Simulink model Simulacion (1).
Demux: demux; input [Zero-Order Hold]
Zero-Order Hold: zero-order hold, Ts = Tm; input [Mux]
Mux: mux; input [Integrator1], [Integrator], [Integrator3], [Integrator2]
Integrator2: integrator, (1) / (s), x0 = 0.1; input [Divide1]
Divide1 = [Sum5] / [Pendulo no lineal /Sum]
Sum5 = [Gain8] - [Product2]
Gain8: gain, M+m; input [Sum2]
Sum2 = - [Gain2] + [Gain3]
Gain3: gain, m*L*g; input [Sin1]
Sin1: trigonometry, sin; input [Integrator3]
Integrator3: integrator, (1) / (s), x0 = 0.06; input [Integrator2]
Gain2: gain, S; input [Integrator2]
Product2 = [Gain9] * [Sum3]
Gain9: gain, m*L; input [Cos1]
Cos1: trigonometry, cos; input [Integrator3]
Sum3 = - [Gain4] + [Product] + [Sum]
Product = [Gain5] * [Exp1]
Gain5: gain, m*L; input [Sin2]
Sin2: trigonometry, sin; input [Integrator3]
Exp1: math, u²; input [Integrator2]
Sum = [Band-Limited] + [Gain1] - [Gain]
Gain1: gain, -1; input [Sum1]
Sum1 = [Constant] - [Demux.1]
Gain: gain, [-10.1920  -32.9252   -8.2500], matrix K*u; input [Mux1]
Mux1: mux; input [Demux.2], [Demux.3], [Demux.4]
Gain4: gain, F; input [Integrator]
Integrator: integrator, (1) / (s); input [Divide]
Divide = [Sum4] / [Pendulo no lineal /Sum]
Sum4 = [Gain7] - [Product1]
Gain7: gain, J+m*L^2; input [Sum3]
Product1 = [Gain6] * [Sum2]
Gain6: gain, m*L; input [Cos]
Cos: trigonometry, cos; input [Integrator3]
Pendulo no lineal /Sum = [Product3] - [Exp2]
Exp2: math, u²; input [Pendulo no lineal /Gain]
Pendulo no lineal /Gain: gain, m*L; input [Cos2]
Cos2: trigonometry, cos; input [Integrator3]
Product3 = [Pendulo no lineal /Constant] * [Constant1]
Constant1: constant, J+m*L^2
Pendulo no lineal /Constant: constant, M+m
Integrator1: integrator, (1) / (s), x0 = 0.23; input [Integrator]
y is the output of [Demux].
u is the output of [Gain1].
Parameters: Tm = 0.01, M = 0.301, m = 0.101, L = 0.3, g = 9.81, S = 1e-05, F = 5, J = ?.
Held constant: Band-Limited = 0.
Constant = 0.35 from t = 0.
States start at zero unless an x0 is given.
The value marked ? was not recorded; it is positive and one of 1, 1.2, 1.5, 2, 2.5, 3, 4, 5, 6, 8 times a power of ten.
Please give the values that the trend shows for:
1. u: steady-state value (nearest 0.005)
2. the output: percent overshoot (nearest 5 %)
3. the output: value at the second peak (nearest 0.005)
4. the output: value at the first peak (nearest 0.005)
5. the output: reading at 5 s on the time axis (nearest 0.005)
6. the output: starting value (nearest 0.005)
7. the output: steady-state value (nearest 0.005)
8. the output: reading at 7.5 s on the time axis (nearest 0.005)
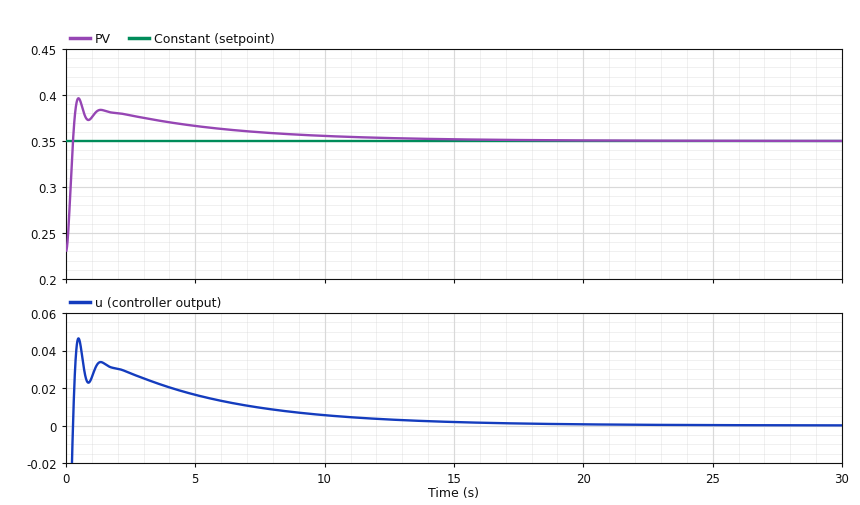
0.000
40 %
0.385
0.395
0.365
0.230
0.350
0.360
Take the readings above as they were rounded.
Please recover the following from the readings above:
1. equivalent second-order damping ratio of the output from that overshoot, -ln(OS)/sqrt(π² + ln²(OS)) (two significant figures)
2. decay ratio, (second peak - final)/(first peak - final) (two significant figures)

0.28
0.78
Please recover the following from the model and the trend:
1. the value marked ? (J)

0.02
